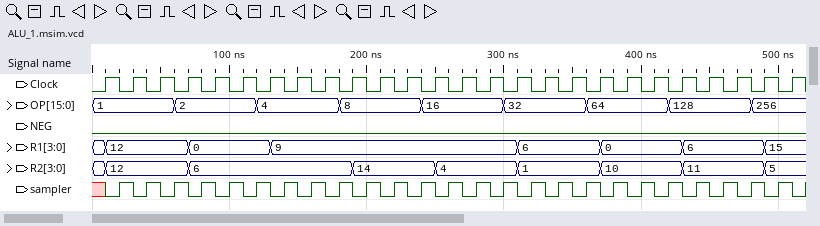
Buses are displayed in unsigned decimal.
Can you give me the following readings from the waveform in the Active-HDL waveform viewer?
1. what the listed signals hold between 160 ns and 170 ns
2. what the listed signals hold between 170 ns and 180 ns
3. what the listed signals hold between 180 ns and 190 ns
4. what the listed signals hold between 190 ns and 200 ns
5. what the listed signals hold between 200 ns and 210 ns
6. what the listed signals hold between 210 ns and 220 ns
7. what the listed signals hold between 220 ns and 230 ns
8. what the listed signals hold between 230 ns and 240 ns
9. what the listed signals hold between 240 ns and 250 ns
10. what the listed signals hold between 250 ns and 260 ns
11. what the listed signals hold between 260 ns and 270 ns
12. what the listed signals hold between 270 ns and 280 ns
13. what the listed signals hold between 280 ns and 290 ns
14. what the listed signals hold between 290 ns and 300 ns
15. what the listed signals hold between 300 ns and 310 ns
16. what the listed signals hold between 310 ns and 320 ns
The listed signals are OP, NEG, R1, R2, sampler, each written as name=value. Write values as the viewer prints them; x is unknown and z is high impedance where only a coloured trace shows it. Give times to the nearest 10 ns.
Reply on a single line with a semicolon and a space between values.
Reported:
OP=4, NEG=0, R1=9, R2=6, sampler=1; OP=4, NEG=0, R1=9, R2=6, sampler=0; OP=8, NEG=0, R1=9, R2=6, sampler=1; OP=8, NEG=0, R1=9, R2=14, sampler=0; OP=8, NEG=0, R1=9, R2=14, sampler=1; OP=8, NEG=0, R1=9, R2=14, sampler=0; OP=8, NEG=0, R1=9, R2=14, sampler=1; OP=8, NEG=0, R1=9, R2=14, sampler=0; OP=16, NEG=0, R1=9, R2=14, sampler=1; OP=16, NEG=0, R1=9, R2=4, sampler=0; OP=16, NEG=0, R1=9, R2=4, sampler=1; OP=16, NEG=0, R1=9, R2=4, sampler=0; OP=16, NEG=0, R1=9, R2=4, sampler=1; OP=16, NEG=0, R1=9, R2=4, sampler=0; OP=32, NEG=0, R1=9, R2=4, sampler=1; OP=32, NEG=0, R1=6, R2=1, sampler=0
